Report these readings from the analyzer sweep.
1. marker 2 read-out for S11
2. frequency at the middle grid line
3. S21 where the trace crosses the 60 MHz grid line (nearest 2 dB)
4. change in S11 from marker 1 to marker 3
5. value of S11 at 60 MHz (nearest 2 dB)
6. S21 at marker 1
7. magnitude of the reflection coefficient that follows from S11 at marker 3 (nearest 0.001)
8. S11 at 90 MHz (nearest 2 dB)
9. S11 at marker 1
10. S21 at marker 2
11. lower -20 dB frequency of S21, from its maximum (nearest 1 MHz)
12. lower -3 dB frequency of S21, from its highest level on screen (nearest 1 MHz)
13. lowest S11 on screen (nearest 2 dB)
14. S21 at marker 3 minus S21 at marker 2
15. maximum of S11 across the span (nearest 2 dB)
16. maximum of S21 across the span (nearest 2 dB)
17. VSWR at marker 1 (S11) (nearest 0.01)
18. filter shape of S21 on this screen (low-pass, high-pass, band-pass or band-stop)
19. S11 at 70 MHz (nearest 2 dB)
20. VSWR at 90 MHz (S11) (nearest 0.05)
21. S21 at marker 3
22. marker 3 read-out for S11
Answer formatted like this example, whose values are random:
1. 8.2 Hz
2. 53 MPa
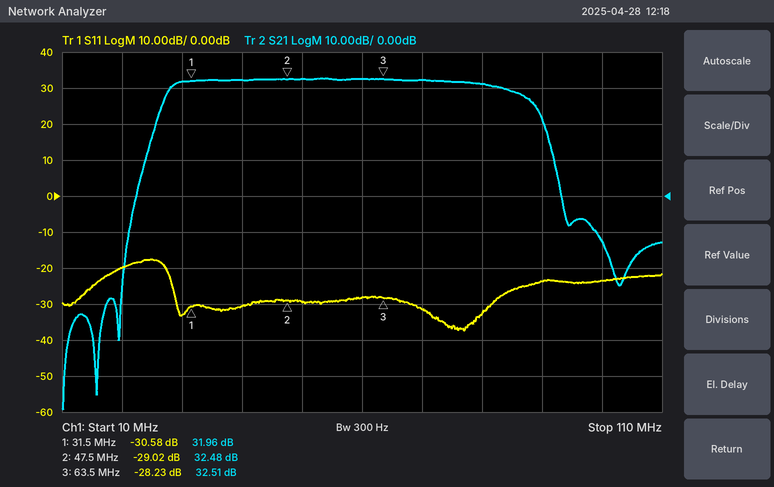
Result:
1. -29.02 dB
2. 60 MHz
3. 32 dB
4. 2.35 dB
5. -28 dB
6. 31.96 dB
7. 0.039
8. -24 dB
9. -30.58 dB
10. 32.48 dB
11. 24 MHz
12. 28 MHz
13. -38 dB
14. 0.03 dB
15. -18 dB
16. 32 dB
17. 1.06
18. band-pass
19. -32 dB
20. 1.15
21. 32.51 dB
22. -28.23 dB
